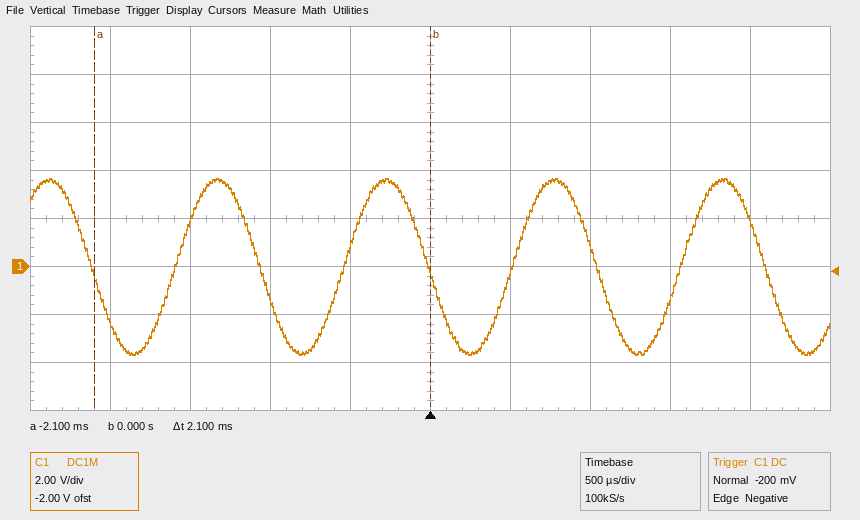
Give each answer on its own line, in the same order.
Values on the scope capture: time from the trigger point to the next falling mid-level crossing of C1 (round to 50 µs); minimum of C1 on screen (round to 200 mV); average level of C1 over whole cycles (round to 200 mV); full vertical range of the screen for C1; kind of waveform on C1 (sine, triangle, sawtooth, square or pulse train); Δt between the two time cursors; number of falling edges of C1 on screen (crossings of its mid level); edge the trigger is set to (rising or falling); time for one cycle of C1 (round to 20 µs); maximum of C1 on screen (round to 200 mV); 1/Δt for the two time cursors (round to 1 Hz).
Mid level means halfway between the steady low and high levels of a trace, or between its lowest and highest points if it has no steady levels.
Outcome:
1.05 ms
-3.6 V
0.0 V
16 V
sine
2.1 ms
5
falling
1.06 ms
3.6 V
476 Hz
